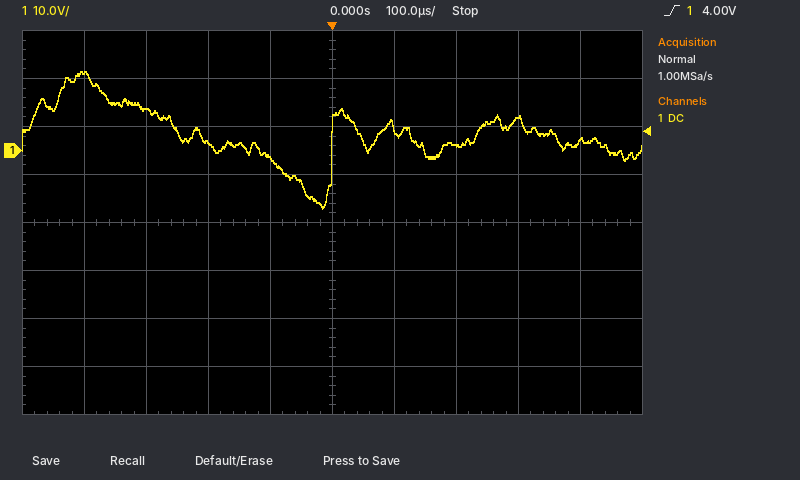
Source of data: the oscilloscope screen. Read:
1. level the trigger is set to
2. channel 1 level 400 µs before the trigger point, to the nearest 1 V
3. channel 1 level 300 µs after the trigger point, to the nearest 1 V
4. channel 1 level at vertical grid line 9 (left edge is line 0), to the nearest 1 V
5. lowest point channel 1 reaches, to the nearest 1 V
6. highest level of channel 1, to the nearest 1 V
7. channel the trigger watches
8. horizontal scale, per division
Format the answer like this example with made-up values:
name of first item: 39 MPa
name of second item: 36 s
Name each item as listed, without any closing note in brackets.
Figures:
level the trigger is set to: 4.00 V
channel 1 level 400 µs before the trigger point, to the nearest 1 V: 16 V
channel 1 level 300 µs after the trigger point, to the nearest 1 V: 7 V
channel 1 level at vertical grid line 9 (left edge is line 0), to the nearest 1 V: 2 V
lowest point channel 1 reaches, to the nearest 1 V: -12 V
highest level of channel 1, to the nearest 1 V: 16 V
channel the trigger watches: channel 1
horizontal scale, per division: 100 µs
